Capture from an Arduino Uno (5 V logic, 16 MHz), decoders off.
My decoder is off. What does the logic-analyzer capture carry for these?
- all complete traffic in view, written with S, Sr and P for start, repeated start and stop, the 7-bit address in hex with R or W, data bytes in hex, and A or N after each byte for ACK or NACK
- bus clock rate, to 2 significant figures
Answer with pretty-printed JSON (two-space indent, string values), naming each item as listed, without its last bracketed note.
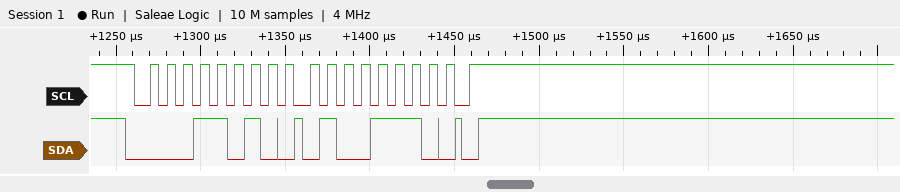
{
  "all complete traffic in view, written with S, Sr and P for start, repeated start and stop, the 7-bit address in hex with R or W, data bytes in hex, and A or N after each byte for ACK or NACK": "S 0DW A 4E A P",
  "bus clock rate, to 2 significant figures": "100 kHz"
}
